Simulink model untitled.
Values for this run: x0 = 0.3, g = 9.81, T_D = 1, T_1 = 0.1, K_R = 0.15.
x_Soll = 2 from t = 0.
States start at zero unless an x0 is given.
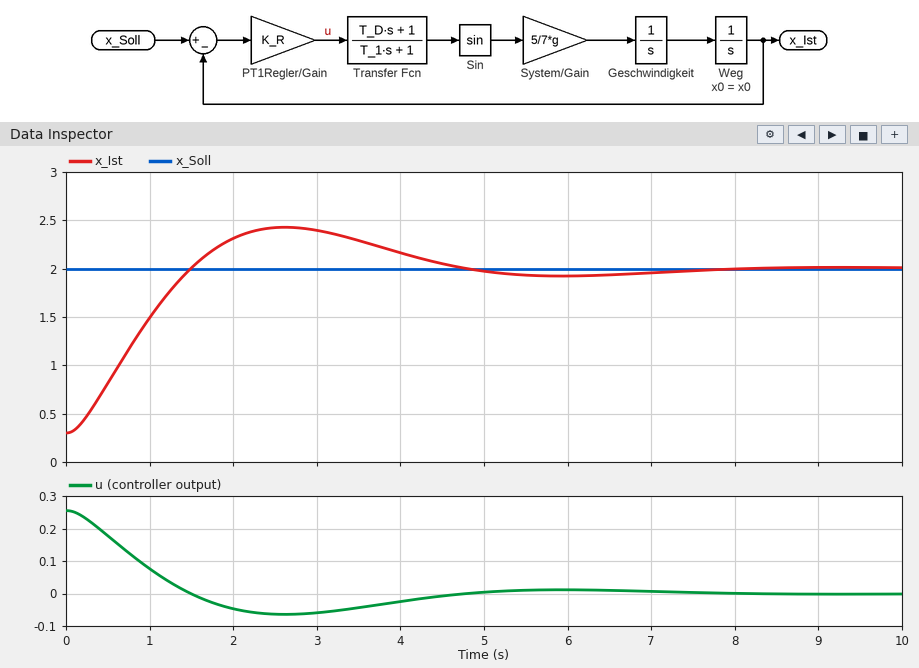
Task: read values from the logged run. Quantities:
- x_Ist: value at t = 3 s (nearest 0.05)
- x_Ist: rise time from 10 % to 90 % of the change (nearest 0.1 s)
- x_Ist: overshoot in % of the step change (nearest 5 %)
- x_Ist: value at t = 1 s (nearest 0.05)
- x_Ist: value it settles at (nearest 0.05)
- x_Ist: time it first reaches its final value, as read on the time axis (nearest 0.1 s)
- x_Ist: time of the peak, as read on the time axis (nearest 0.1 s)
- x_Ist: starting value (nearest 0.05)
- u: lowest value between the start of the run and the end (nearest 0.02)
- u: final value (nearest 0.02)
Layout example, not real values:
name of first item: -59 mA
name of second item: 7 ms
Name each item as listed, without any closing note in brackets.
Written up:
x_Ist: value at t = 3 s: 2.40
x_Ist: rise time from 10 % to 90 % of the change: 1.1 s
x_Ist: overshoot in % of the step change: 25 %
x_Ist: value at t = 1 s: 1.50
x_Ist: value it settles at: 2.00
x_Ist: time it first reaches its final value, as read on the time axis: 1.5 s
x_Ist: time of the peak, as read on the time axis: 2.6 s
x_Ist: starting value: 0.30
u: lowest value between the start of the run and the end: -0.06
u: final value: 0.00
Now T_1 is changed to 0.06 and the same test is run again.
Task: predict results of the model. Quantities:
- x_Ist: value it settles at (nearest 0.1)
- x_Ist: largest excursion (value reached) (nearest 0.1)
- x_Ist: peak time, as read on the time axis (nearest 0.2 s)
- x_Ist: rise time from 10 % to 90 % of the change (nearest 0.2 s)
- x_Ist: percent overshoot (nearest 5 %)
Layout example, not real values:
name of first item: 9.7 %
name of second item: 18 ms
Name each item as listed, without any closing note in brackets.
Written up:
x_Ist: value it settles at: 2.0
x_Ist: largest excursion (value reached): 2.3
x_Ist: peak time, as read on the time axis: 3.0 s
x_Ist: rise time from 10 % to 90 % of the change: 1.4 s
x_Ist: percent overshoot: 20 %
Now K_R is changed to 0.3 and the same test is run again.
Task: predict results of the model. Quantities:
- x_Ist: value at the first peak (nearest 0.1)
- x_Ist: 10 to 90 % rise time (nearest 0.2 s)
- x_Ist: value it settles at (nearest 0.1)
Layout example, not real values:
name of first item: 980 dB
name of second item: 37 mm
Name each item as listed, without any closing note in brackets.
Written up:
x_Ist: value at the first peak: 2.1
x_Ist: 10 to 90 % rise time: 1.2 s
x_Ist: value it settles at: 2.0
